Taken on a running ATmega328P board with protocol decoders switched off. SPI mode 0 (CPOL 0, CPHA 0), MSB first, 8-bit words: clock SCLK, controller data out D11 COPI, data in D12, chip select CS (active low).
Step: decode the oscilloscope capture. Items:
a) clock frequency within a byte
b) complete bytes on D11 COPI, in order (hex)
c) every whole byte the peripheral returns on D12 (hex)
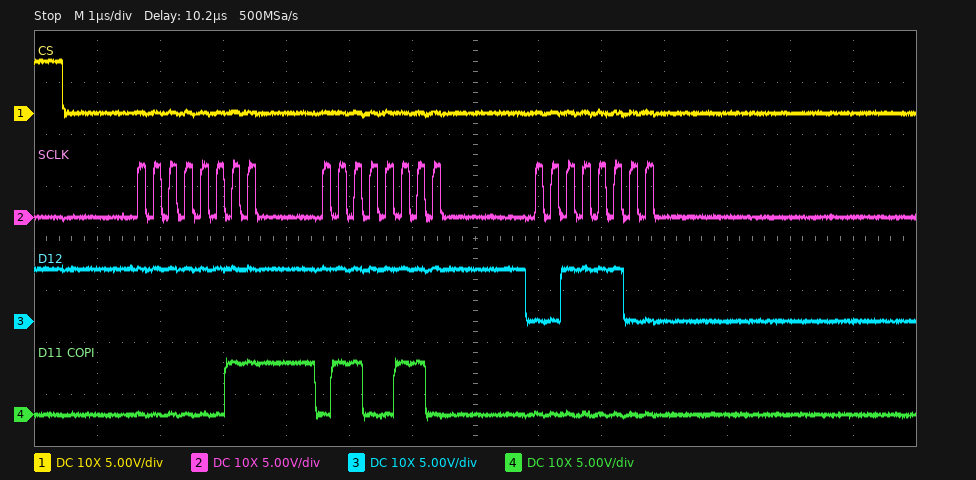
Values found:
4 MHz
0x03 0x66 0x00
0xFF 0xFF 0x3C
